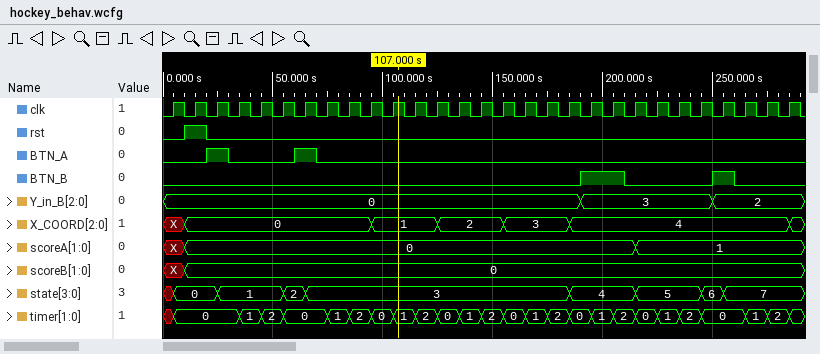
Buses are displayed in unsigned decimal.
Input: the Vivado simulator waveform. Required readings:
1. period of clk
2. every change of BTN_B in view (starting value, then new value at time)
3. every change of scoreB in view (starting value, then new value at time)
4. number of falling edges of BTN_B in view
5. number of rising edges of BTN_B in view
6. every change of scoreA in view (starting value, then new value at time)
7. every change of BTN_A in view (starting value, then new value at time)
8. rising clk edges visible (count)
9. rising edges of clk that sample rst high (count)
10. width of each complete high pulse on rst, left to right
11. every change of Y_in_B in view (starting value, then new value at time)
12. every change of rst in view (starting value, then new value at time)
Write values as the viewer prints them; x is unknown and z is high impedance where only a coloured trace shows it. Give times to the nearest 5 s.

10 s
0, 1 at 190 s, 0 at 210 s, 1 at 250 s, 0 at 260 s
X, 0 at 10 s
2
2
X, 0 at 10 s, 1 at 215 s
0, 1 at 20 s, 0 at 30 s, 1 at 60 s, 0 at 70 s
29
1
10 s
0, 3 at 190 s, 2 at 250 s
0, 1 at 10 s, 0 at 20 s
